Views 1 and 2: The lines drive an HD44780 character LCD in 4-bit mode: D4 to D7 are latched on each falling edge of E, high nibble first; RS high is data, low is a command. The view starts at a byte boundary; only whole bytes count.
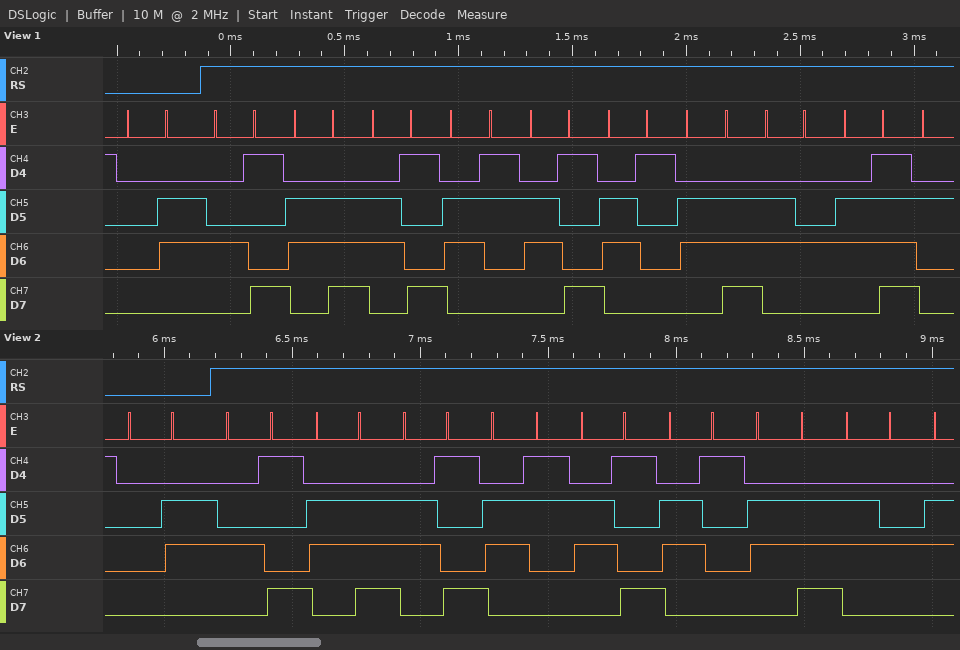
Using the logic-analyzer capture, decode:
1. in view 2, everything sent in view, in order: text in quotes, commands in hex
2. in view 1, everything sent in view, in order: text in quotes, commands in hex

0x06 "Iniciand"
0x06 "Iniciando"
